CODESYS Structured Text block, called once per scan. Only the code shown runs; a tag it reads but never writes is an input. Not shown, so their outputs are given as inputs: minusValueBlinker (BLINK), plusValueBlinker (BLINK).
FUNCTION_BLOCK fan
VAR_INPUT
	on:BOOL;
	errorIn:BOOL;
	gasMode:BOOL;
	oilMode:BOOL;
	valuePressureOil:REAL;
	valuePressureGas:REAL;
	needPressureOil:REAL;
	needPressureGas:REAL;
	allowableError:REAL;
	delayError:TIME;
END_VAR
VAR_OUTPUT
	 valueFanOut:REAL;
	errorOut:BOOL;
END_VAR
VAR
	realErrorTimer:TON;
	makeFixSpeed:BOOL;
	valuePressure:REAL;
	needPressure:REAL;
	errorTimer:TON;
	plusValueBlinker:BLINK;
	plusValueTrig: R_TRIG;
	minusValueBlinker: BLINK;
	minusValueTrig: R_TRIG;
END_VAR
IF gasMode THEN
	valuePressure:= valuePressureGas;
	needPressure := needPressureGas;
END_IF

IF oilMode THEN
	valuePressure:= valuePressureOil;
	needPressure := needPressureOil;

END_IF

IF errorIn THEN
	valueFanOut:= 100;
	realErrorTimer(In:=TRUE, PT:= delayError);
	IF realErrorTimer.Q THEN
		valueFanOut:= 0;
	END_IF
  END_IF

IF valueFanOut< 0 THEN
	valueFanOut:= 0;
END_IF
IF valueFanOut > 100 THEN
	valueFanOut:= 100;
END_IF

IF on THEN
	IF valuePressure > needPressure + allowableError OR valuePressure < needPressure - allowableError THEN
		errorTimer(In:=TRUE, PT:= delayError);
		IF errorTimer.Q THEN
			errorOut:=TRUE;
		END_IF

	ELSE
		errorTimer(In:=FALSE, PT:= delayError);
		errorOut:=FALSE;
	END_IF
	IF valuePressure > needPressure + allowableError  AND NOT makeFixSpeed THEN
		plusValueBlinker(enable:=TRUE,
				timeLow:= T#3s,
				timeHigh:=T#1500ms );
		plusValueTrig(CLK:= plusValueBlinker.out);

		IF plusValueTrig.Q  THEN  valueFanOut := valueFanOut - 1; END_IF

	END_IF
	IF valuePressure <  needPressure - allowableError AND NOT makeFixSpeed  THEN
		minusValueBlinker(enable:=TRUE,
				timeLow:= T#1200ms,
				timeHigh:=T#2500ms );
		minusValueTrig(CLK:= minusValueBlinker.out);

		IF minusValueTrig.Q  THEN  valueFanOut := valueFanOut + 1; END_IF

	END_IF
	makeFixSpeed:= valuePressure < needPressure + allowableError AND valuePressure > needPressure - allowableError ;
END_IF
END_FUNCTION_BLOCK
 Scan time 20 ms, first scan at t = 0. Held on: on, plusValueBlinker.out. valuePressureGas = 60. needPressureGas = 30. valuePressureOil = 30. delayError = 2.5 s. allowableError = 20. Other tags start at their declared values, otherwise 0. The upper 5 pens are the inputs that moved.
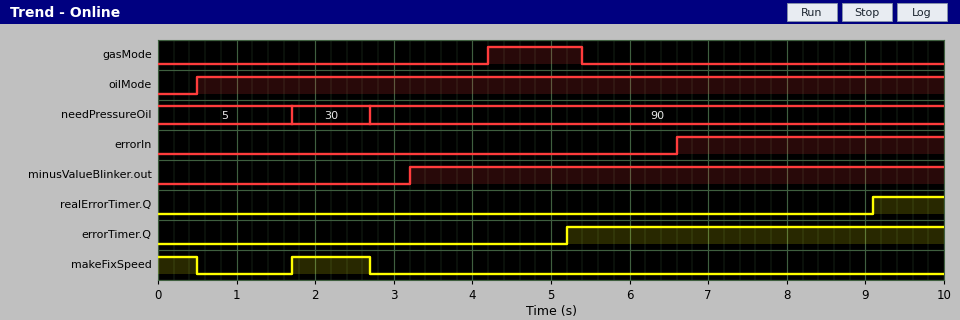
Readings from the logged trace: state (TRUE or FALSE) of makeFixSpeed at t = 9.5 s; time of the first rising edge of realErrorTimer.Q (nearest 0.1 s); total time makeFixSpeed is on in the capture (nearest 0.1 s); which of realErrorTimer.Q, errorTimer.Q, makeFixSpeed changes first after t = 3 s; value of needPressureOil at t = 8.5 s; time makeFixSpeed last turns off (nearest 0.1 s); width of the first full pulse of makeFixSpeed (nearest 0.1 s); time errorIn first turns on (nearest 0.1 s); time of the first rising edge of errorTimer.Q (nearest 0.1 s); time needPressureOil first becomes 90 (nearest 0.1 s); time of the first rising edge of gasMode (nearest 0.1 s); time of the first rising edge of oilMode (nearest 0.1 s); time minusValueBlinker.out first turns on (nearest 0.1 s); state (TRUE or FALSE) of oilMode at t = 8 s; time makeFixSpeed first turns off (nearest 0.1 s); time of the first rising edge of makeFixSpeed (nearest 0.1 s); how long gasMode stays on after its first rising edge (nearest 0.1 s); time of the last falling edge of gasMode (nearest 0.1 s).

FALSE
9.1 s
1.5 s
errorTimer.Q
90
2.7 s
1.0 s
6.6 s
5.2 s
2.7 s
4.2 s
0.5 s
3.2 s
TRUE
0.5 s
1.7 s
1.2 s
5.4 s
